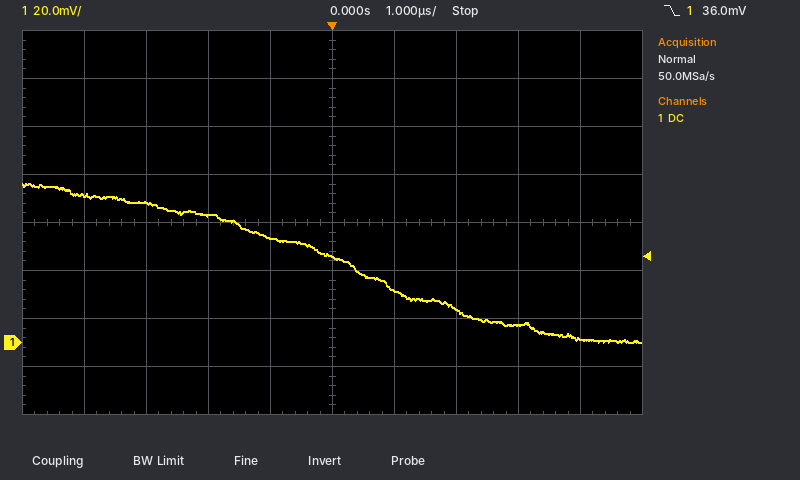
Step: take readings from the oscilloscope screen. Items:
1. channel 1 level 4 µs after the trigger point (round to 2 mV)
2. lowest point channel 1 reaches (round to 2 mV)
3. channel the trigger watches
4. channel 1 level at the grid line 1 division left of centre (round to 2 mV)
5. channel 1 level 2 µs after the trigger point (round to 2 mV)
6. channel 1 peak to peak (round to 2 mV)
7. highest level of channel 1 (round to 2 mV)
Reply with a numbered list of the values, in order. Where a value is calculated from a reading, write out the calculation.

1. 2 mV
2. 0 mV
3. channel 1
4. 44 mV
5. 14 mV
6. 66 mV − (0 mV) = 66 mV
7. 66 mV
